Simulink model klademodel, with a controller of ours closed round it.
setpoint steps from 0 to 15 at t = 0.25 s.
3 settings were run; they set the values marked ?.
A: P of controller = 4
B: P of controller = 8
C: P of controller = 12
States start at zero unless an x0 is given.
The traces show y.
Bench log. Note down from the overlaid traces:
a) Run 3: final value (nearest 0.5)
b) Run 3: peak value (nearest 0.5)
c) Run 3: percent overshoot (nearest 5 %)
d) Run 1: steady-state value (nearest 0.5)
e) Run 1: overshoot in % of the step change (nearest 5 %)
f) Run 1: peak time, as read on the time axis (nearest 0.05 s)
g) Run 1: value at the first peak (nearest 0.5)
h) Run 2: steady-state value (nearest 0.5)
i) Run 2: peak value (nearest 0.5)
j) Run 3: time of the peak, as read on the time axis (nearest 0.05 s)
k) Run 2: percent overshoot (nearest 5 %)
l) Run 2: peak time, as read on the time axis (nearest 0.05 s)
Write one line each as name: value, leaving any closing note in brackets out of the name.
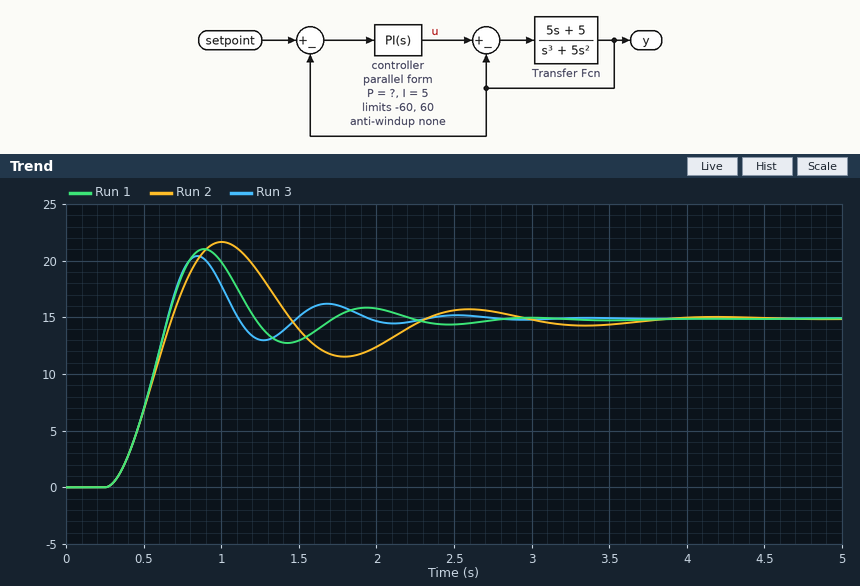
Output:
Run 3: final value: 15.0
Run 3: peak value: 20.5
Run 3: percent overshoot: 35 %
Run 1: steady-state value: 15.0
Run 1: overshoot in % of the step change: 40 %
Run 1: peak time, as read on the time axis: 0.90 s
Run 1: value at the first peak: 21.0
Run 2: steady-state value: 15.0
Run 2: peak value: 21.5
Run 3: time of the peak, as read on the time axis: 0.85 s
Run 2: percent overshoot: 45 %
Run 2: peak time, as read on the time axis: 1.00 s
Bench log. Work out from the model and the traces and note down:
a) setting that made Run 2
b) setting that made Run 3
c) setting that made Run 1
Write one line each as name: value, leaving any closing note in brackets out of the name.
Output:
setting that made Run 2: A
setting that made Run 3: C
setting that made Run 1: B
